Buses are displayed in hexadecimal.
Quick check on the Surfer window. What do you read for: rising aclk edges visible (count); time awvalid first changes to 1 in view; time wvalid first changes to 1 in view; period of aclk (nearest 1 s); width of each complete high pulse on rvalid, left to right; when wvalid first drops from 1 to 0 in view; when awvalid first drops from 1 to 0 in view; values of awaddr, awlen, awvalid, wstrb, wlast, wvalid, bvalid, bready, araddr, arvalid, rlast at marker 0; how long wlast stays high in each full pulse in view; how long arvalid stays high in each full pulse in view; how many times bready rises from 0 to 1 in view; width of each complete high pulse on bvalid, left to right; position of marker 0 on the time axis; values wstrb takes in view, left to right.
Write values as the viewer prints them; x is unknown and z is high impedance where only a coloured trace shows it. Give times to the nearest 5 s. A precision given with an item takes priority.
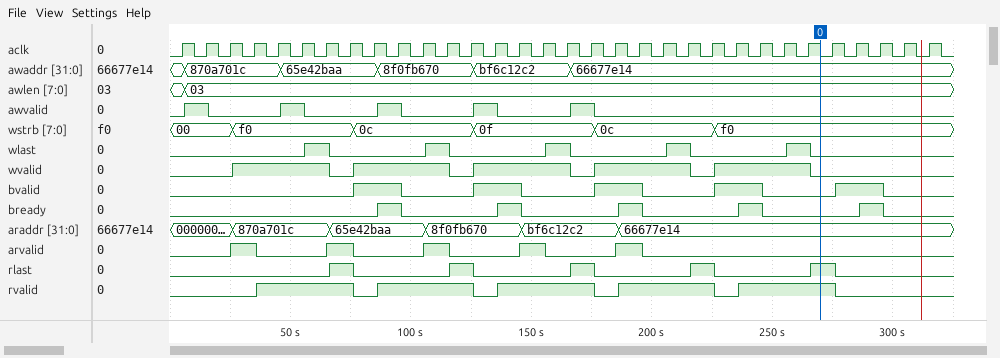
32
5 s
25 s
10 s
40 s, 40 s, 40 s, 40 s, 40 s
65 s
15 s
awaddr=66677e14, awlen=03, awvalid=0, wstrb=f0, wlast=0, wvalid=0, bvalid=0, bready=0, araddr=66677e14, arvalid=0, rlast=1
10 s, 10 s, 10 s, 10 s, 10 s
10 s, 10 s, 10 s, 10 s, 10 s
5
20 s, 20 s, 20 s, 20 s, 20 s
270 s
00, f0, 0c, 0f, 0c, f0
